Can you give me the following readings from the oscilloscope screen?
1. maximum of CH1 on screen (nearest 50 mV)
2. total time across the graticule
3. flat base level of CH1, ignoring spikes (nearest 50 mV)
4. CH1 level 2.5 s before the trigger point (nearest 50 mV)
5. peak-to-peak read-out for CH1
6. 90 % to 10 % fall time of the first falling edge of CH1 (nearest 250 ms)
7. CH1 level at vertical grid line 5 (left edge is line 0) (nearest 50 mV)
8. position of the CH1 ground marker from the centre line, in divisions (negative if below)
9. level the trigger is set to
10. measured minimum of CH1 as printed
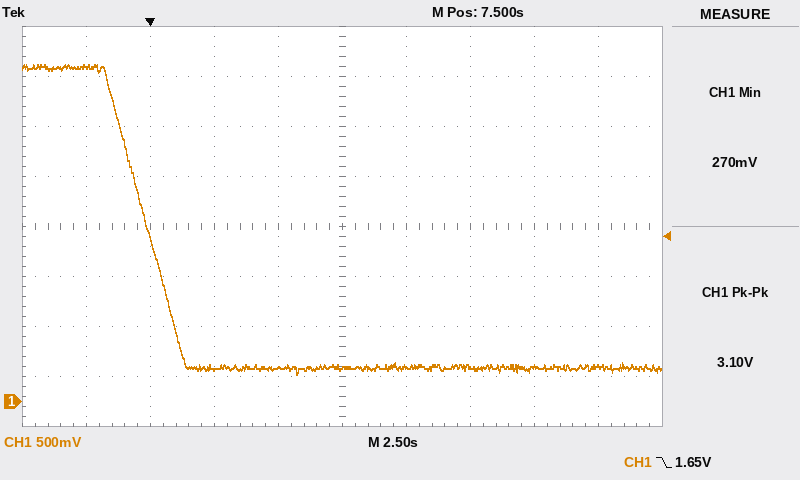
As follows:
3.35 V
25 s
350 mV
3.35 V
3.10 V
2.50 s
350 mV
-3.5 div
1.65 V
270 mV
